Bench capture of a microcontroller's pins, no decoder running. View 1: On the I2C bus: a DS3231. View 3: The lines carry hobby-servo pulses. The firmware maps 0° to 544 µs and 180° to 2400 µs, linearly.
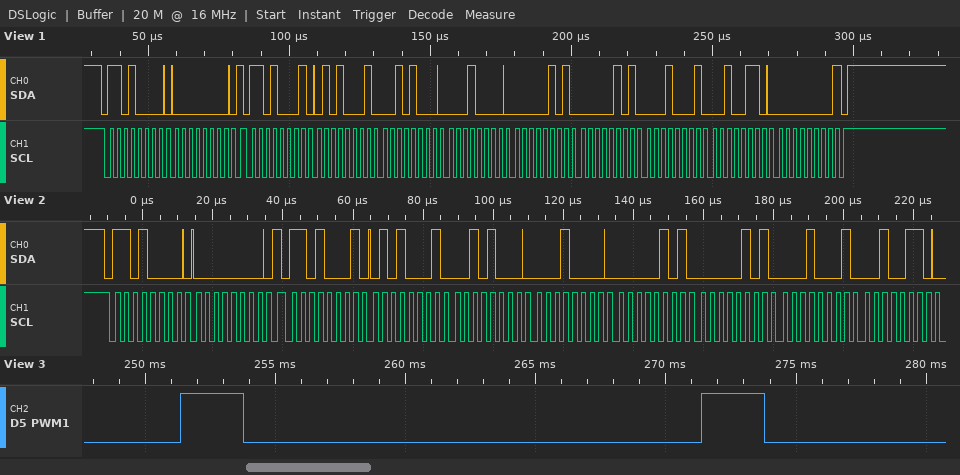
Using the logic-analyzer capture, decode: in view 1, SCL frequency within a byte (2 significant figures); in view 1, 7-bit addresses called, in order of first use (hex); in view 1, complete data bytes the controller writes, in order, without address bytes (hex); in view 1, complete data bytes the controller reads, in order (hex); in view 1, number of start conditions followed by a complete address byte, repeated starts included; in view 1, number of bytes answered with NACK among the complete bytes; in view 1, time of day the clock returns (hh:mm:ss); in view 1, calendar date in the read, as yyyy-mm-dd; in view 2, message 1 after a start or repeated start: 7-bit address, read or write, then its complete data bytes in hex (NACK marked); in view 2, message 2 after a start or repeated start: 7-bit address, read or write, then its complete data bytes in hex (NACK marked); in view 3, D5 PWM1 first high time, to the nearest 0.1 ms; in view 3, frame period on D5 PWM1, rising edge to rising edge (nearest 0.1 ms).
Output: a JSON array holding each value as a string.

["400 kHz", "0x68", "00", "51 28 10 05 05 11 26 00", "2", "1", "10:28:51", "2026-11-05", "0x68 write: 00", "0x68 read: 51 28 10 05 05 11 26", "2.4 ms", "20.0 ms"]
